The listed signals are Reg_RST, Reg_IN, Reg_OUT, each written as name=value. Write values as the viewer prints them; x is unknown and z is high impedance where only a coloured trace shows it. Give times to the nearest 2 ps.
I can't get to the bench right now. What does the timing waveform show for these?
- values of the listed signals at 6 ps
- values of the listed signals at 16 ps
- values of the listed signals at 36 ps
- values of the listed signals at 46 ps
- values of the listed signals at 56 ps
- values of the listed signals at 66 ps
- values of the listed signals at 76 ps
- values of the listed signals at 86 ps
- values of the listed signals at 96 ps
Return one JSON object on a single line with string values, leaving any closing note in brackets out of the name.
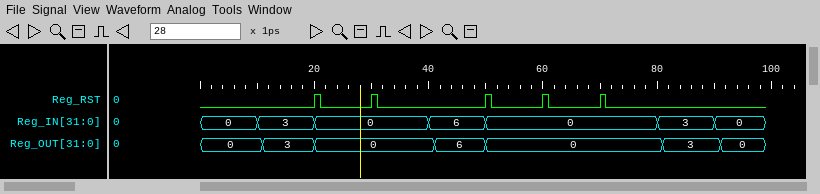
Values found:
{"values of the listed signals at 6 ps": "Reg_RST=0, Reg_IN=0, Reg_OUT=0", "values of the listed signals at 16 ps": "Reg_RST=0, Reg_IN=3, Reg_OUT=3", "values of the listed signals at 36 ps": "Reg_RST=0, Reg_IN=0, Reg_OUT=0", "values of the listed signals at 46 ps": "Reg_RST=0, Reg_IN=6, Reg_OUT=6", "values of the listed signals at 56 ps": "Reg_RST=0, Reg_IN=0, Reg_OUT=0", "values of the listed signals at 66 ps": "Reg_RST=0, Reg_IN=0, Reg_OUT=0", "values of the listed signals at 76 ps": "Reg_RST=0, Reg_IN=0, Reg_OUT=0", "values of the listed signals at 86 ps": "Reg_RST=0, Reg_IN=3, Reg_OUT=3", "values of the listed signals at 96 ps": "Reg_RST=0, Reg_IN=0, Reg_OUT=0"}
